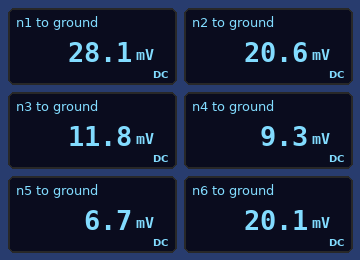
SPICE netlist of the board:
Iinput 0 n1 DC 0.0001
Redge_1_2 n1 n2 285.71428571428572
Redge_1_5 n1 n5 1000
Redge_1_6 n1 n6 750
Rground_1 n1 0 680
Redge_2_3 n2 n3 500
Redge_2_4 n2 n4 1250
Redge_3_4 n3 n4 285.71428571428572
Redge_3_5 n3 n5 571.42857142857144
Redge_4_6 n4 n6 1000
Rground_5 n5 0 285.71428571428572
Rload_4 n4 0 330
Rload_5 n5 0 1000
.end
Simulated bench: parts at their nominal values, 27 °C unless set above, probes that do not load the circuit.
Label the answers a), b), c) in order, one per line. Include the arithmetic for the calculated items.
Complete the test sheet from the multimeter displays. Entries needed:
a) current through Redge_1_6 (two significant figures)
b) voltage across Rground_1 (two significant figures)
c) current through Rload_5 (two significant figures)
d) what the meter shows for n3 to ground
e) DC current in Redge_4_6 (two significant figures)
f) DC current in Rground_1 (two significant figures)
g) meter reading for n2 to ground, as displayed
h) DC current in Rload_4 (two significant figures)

a) (28.1 mV - 20.1 mV) / 750 Ω = 11 µA
b) 28.1 mV = 28 mV
c) (6.7 mV) / 1 kΩ = 6.7 µA
d) 11.8 mV
e) (20.1 mV - 9.3 mV) / 1 kΩ = 11 µA
f) (28.1 mV) / 680 Ω = 41 µA
g) 20.6 mV
h) (9.3 mV) / 330 Ω = 28 µA
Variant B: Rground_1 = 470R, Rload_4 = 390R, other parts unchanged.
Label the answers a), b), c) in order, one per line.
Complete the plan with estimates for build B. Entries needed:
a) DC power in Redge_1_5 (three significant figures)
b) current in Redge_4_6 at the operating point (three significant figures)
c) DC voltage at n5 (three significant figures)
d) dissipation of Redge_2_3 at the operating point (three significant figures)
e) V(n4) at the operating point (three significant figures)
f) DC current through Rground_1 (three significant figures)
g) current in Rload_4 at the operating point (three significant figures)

a) 331 nW
b) 8.76 µA
c) 5.87 mV
d) 106 nW
e) 8.73 mV
f) 51.2 µA
g) 22.4 µA
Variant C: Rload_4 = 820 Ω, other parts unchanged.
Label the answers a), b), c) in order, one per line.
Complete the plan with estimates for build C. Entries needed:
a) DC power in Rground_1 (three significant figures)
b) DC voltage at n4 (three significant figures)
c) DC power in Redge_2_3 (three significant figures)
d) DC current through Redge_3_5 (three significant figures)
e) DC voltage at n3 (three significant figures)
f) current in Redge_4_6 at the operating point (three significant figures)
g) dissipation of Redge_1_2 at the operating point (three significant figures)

a) 1.39 µW
b) 15.2 mV
c) 132 nW
d) 13.7 µA
e) 15.9 mV
f) 8.87 µA
g) 156 nW
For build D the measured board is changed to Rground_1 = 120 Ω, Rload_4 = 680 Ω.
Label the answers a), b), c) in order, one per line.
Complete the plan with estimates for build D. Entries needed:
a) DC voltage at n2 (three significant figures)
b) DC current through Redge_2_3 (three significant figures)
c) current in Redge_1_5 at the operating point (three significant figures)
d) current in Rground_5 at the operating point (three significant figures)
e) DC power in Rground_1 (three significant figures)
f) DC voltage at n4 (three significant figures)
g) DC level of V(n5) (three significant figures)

a) 7.59 mV
b) 5.38 µA
c) 7.29 µA
d) 8.89 µA
e) 805 nW
f) 4.55 mV
g) 2.54 mV
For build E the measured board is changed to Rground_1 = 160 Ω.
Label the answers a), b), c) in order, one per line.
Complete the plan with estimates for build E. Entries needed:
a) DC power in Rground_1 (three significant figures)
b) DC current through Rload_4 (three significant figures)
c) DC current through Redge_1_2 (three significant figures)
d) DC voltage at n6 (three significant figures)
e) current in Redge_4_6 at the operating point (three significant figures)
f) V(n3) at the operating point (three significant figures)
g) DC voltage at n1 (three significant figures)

a) 900 nW
b) 12.1 µA
c) 11.3 µA
d) 8.57 mV
e) 4.58 µA
f) 5.04 mV
g) 12.0 mV
